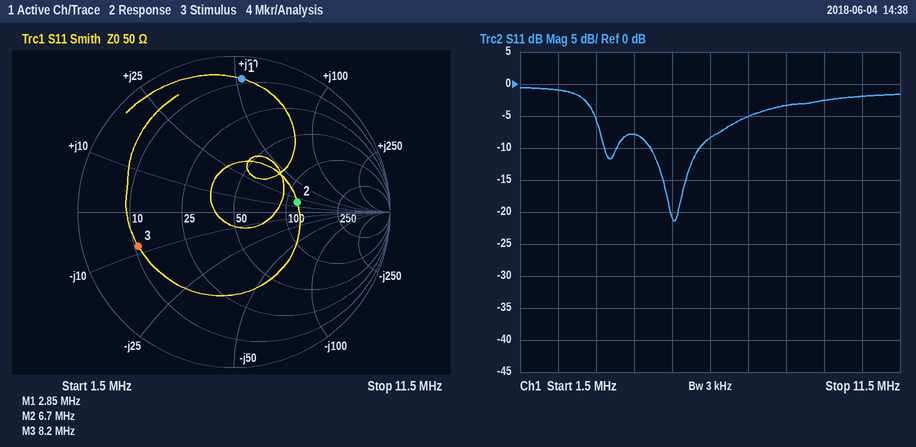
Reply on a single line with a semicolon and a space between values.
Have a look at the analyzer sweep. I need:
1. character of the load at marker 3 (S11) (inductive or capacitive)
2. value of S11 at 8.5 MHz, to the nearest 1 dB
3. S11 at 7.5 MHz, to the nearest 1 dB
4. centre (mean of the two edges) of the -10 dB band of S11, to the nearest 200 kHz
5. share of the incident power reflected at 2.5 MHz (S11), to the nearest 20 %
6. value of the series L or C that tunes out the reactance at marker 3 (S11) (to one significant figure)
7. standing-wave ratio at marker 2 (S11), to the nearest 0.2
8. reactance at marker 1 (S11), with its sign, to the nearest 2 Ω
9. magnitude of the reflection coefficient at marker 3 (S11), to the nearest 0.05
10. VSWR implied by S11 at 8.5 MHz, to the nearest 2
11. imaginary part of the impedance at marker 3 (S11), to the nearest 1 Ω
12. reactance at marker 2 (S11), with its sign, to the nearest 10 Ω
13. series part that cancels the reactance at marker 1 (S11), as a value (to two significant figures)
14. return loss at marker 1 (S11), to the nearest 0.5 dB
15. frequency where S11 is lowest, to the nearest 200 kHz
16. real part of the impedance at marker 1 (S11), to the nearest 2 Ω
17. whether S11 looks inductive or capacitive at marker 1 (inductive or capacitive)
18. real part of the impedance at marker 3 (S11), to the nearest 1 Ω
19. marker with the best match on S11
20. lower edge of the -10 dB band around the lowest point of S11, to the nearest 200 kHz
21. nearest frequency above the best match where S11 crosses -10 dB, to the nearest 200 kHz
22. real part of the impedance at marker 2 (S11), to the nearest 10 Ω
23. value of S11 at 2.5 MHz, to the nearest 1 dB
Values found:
capacitive; -3 dB; -5 dB; 5.6 MHz; 80 %; 200 nH; 2.4; +52 Ω; 0.65; 6; -8 Ω; +20 Ω; 1.1 nF; 1.5 dB; 5.6 MHz; 8 Ω; inductive; 11 Ω; marker 2; 5.0 MHz; 6.2 MHz; 120 Ω; -1 dB
